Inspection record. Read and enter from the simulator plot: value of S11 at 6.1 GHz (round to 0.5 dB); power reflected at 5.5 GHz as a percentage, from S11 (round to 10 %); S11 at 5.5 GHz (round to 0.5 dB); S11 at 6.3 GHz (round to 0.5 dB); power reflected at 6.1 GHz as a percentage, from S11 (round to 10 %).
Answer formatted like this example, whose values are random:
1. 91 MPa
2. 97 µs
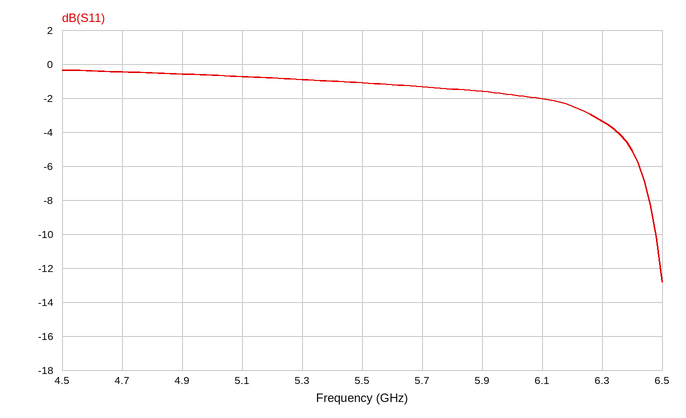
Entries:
1. -2.0 dB
2. 80 %
3. -1.0 dB
4. -3.5 dB
5. 60 %
